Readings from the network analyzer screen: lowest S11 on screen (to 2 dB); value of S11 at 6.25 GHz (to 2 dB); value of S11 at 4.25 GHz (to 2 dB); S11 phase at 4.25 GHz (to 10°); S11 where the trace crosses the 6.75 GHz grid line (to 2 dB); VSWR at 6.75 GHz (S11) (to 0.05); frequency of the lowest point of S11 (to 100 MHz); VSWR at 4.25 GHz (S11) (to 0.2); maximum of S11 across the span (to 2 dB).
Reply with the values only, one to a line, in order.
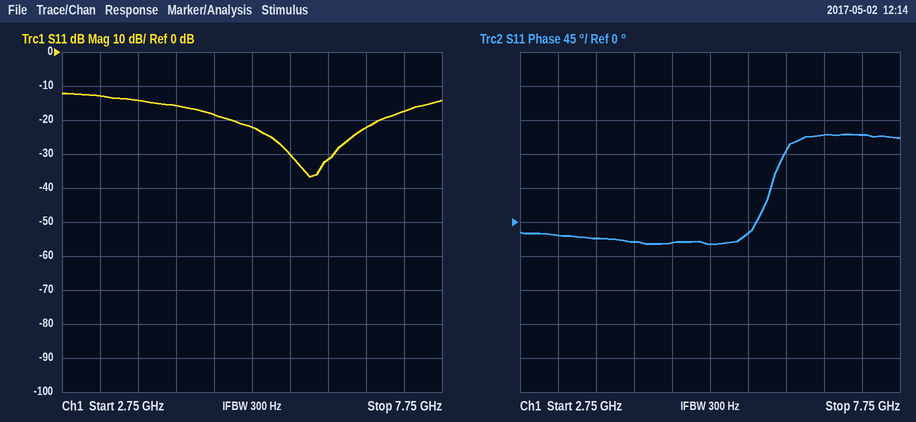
-36 dB
-32 dB
-16 dB
-30°
-22 dB
1.15
6.0 GHz
1.4
-12 dB
